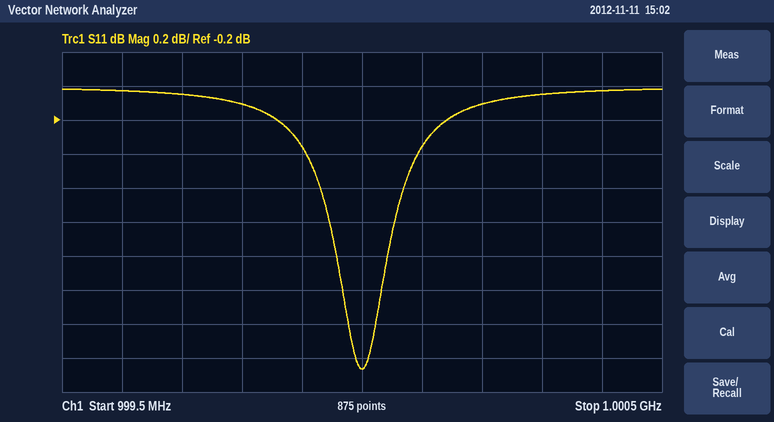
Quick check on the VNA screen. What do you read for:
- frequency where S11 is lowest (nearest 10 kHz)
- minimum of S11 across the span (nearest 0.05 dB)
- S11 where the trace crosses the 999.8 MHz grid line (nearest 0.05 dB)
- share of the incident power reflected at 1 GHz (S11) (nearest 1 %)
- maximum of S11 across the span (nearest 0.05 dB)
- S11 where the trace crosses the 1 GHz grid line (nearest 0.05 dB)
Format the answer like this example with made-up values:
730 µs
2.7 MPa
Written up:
1.00000 GHz
-1.65 dB
-0.10 dB
68 %
0.00 dB
-1.65 dB
